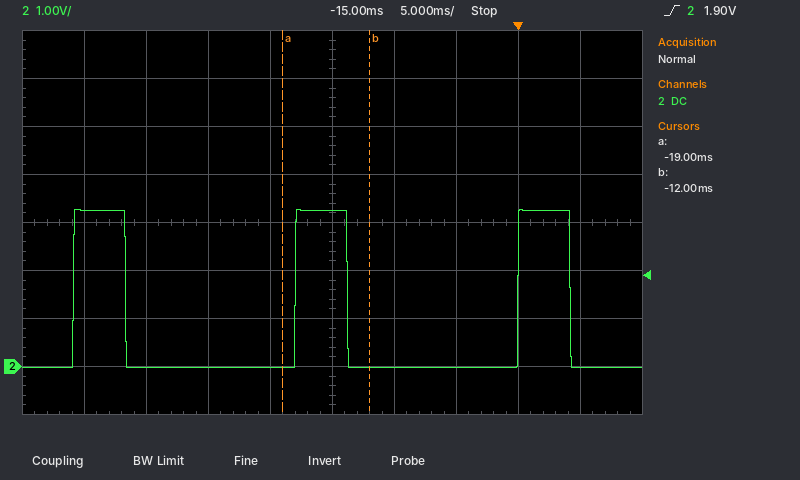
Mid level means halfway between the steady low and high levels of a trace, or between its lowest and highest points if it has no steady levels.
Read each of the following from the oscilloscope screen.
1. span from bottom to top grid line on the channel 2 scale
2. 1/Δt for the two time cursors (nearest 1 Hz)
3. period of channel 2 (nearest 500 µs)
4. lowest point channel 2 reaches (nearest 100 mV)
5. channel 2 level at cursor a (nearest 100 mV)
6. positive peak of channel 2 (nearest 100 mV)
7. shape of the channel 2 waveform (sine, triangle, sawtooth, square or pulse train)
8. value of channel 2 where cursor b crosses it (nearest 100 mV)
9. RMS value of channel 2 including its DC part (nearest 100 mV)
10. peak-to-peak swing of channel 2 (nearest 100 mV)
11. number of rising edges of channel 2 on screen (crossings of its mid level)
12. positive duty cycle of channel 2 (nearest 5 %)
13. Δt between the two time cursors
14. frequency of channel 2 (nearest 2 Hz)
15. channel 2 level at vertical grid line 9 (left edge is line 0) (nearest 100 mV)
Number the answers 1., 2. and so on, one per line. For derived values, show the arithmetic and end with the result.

1. 8 V
2. 1 / 7.0 ms ≈ 143 Hz
3. 18.0 ms
4. 0.0 V
5. 0.0 V
6. 3.3 V
7. pulse train
8. 0.0 V
9. √(0.25 × (3.3 V)² + 0.75 × (0.0 V)²) ≈ 1.6 V
10. 3.3 V − (0.0 V) = 3.3 V
11. 3
12. 25 %
13. -12 ms − (-19 ms) = 7.0 ms
14. 1 / 18.0 ms ≈ 56 Hz
15. 0.0 V
